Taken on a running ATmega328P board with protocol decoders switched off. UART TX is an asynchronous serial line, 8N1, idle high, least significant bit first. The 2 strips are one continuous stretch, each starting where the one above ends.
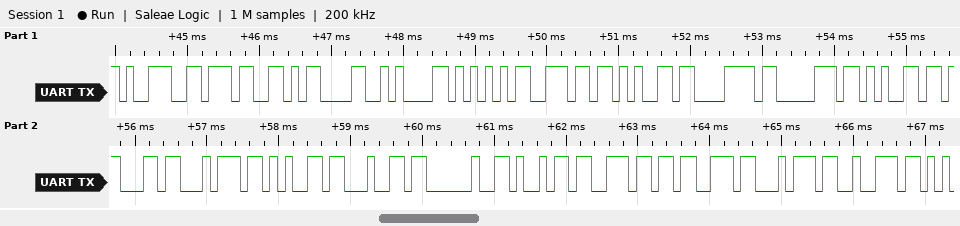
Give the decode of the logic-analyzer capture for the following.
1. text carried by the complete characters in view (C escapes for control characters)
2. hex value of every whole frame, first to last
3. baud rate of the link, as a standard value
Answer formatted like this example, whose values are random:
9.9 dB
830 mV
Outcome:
"97\r\nUnexpected instr"
39 37 0D 0A 55 6E 65 78 70 65 63 74 65 64 20 69 6E 73 74 72
9600 baud
